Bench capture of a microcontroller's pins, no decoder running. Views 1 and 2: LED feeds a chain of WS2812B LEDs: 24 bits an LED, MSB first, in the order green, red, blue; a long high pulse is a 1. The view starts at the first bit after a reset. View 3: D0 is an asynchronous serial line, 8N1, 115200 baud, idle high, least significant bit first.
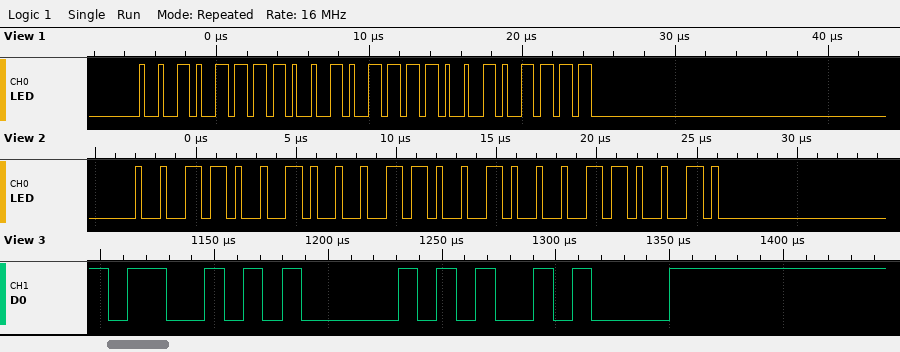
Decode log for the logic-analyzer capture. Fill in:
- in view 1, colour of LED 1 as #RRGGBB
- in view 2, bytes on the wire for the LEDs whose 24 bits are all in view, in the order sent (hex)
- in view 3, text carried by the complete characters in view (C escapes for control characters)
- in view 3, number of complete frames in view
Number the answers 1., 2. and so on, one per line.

1. #2F2F2F
2. 32 32 32
3. "SP\n"
4. 3
